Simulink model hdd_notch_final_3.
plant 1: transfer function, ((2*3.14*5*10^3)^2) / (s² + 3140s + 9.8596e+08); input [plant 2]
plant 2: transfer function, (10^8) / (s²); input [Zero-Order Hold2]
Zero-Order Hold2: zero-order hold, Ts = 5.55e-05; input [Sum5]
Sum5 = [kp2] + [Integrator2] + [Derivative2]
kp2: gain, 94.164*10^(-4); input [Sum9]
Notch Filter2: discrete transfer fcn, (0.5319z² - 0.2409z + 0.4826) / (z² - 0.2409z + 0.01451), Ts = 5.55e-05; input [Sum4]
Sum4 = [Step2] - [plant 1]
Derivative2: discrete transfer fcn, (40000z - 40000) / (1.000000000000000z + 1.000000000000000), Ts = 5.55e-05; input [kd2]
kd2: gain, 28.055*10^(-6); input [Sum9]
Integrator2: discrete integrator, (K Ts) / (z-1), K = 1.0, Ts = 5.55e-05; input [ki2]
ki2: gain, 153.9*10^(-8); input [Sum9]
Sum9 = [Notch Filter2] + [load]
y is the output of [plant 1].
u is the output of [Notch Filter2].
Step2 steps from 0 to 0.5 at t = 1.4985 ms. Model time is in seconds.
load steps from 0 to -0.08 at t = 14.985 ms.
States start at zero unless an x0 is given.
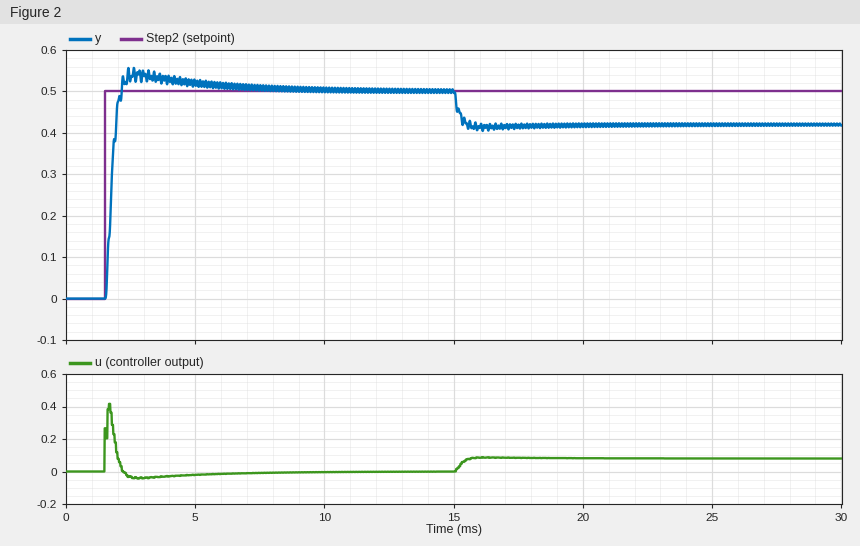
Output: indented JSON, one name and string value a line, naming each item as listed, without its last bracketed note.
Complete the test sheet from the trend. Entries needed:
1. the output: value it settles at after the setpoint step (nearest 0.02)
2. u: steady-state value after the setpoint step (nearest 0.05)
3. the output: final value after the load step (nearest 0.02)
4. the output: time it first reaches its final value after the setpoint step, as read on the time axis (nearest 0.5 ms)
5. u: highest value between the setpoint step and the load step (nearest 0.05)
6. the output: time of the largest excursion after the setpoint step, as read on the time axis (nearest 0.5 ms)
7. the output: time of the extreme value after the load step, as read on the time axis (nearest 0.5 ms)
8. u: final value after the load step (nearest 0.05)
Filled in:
{
  "the output: value it settles at after the setpoint step": "0.50",
  "u: steady-state value after the setpoint step": "0.00",
  "the output: final value after the load step": "0.42",
  "the output: time it first reaches its final value after the setpoint step, as read on the time axis": "2.0 ms",
  "u: highest value between the setpoint step and the load step": "0.40",
  "the output: time of the largest excursion after the setpoint step, as read on the time axis": "2.5 ms",
  "the output: time of the extreme value after the load step, as read on the time axis": "16.0 ms",
  "u: final value after the load step": "0.10"
}
